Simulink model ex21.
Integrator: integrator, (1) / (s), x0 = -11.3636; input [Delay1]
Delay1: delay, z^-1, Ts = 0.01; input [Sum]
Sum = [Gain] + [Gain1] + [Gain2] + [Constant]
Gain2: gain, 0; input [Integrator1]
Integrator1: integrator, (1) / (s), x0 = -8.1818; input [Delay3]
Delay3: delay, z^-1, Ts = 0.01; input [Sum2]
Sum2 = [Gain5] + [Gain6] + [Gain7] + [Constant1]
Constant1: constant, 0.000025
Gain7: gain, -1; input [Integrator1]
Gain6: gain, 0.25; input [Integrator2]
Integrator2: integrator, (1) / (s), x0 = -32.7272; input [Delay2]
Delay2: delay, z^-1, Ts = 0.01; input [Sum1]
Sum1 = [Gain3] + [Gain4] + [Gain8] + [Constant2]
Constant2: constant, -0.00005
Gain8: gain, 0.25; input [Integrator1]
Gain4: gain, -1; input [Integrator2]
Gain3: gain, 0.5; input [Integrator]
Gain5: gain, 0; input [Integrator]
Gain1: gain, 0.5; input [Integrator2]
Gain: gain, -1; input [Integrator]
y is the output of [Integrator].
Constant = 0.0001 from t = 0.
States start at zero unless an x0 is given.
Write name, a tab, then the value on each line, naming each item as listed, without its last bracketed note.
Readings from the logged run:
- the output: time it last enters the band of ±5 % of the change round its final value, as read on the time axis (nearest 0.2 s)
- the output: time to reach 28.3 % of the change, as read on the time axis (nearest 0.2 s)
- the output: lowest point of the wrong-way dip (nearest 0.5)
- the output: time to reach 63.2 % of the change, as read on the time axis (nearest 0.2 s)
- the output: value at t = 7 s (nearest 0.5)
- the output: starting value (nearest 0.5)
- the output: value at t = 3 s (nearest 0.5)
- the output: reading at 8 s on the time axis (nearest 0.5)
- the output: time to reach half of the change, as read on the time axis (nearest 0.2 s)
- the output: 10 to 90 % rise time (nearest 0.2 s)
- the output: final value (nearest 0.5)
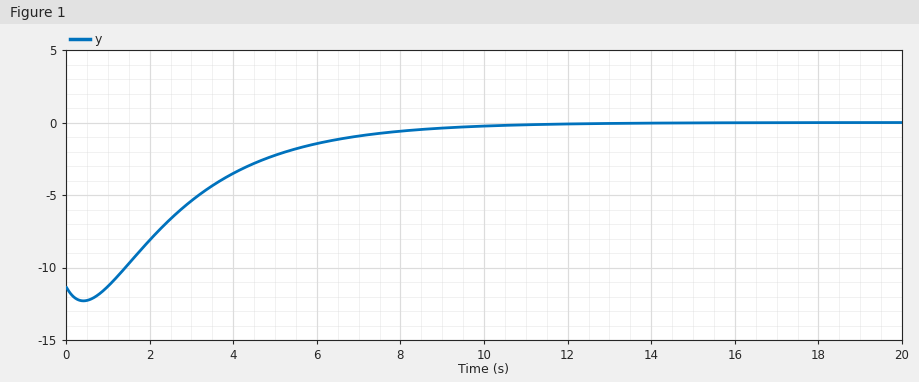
the output: time it last enters the band of ±5 % of the change round its final value, as read on the time axis	8.2 s
the output: time to reach 28.3 % of the change, as read on the time axis	2.0 s
the output: lowest point of the wrong-way dip	-12.5
the output: time to reach 63.2 % of the change, as read on the time axis	3.6 s
the output: value at t = 7 s	-1.0
the output: starting value	-11.5
the output: value at t = 3 s	-5.5
the output: reading at 8 s on the time axis	-0.5
the output: time to reach half of the change, as read on the time axis	2.8 s
the output: 10 to 90 % rise time	5.2 s
the output: final value	0.0
